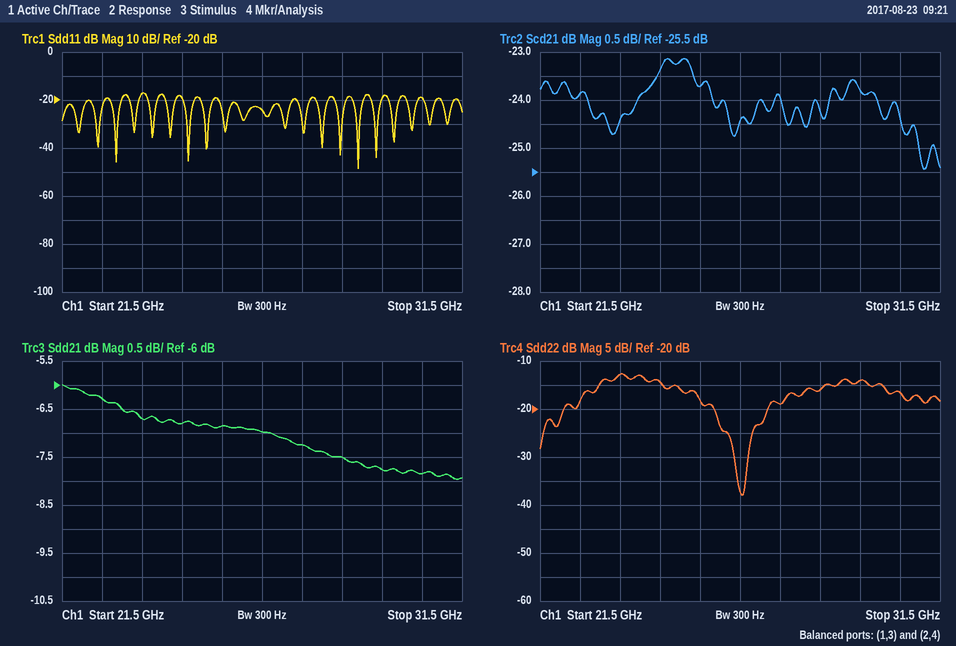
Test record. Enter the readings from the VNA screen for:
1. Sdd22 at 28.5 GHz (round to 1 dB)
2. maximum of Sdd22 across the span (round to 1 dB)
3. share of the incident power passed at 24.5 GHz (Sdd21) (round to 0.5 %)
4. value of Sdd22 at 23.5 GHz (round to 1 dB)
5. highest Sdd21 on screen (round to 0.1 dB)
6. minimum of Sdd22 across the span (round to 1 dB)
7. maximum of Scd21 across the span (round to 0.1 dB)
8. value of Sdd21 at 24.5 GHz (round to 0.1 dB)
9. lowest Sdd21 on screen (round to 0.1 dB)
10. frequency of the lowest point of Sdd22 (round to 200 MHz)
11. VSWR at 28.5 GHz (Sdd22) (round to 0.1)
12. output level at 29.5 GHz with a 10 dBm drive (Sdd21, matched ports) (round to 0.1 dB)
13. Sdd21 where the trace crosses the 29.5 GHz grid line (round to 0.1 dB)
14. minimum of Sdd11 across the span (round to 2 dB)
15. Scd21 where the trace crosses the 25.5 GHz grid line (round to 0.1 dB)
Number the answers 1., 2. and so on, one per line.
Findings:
1. -16 dB
2. -13 dB
3. 21.0 %
4. -13 dB
5. -6.0 dB
6. -38 dB
7. -23.1 dB
8. -6.8 dB
9. -8.0 dB
10. 26.6 GHz
11. 1.4
12. 2.2 dBm
13. -7.8 dB
14. -48 dB
15. -23.7 dB
